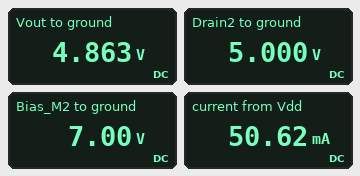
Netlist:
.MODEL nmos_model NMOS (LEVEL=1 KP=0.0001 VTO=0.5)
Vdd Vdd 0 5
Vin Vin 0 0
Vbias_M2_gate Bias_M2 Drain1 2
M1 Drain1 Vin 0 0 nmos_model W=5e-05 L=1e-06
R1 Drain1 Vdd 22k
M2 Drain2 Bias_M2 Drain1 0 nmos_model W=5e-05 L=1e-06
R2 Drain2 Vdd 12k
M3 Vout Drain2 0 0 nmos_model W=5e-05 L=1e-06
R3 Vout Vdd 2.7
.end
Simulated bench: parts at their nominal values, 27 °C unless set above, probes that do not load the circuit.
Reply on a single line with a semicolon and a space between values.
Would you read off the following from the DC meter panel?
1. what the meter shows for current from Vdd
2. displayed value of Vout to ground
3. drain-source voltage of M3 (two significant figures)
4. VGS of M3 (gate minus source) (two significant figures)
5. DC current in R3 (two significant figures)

50.62 mA; 4.863 V; 4.9 V; 5.0 V; 51 mA
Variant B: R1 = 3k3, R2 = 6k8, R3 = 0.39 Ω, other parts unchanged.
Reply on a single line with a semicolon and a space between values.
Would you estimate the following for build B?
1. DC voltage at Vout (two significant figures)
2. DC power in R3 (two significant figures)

5.0 V; 1.0 mW
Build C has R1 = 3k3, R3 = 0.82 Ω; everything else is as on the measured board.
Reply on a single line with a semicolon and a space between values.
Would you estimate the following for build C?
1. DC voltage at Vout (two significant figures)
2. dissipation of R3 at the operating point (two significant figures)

5.0 V; 2.1 mW
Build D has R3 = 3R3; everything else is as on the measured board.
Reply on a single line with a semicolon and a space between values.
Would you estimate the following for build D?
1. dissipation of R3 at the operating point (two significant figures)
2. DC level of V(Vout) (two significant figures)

8.5 mW; 4.8 V
